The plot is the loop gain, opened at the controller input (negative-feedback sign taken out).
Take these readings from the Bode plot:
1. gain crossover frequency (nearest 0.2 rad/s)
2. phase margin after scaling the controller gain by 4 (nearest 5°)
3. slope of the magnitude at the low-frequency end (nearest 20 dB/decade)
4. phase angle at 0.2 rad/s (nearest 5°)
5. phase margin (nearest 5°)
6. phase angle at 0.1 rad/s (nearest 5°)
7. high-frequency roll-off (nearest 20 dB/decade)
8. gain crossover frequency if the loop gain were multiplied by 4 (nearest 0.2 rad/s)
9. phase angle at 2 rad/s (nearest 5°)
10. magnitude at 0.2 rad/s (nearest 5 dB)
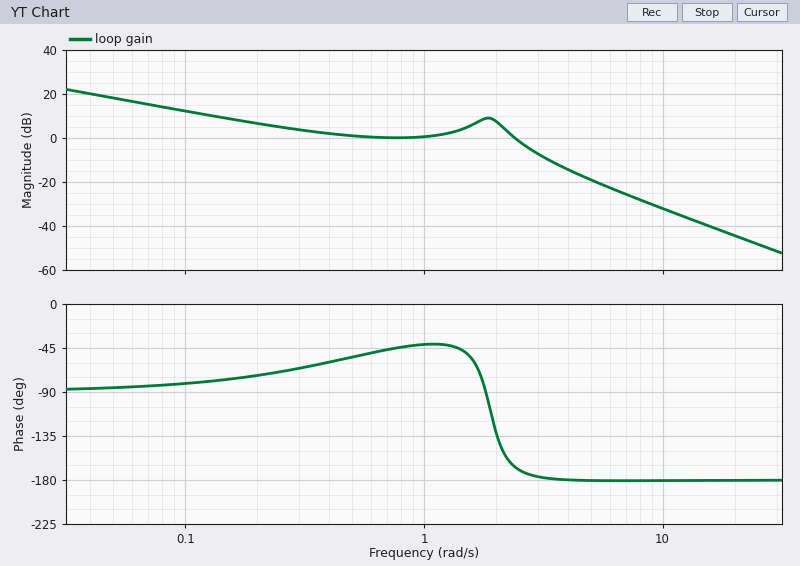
2.4 rad/s
0°
-20 dB/decade
-75°
15°
-80°
-40 dB/decade
3.6 rad/s
-130°
5 dB
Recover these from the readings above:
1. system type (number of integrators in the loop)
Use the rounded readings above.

1
